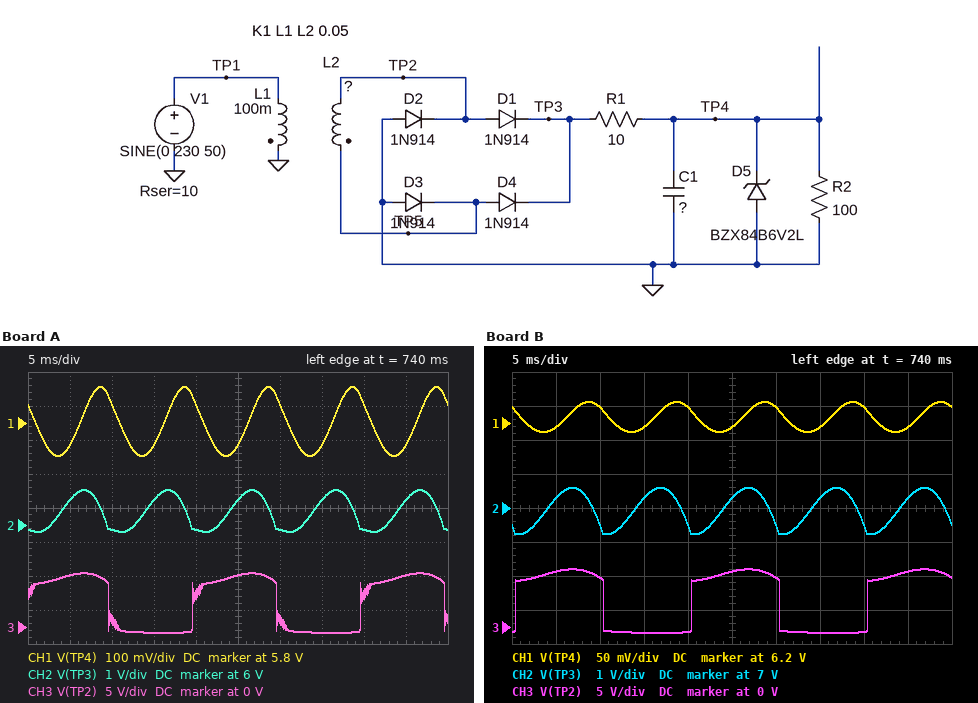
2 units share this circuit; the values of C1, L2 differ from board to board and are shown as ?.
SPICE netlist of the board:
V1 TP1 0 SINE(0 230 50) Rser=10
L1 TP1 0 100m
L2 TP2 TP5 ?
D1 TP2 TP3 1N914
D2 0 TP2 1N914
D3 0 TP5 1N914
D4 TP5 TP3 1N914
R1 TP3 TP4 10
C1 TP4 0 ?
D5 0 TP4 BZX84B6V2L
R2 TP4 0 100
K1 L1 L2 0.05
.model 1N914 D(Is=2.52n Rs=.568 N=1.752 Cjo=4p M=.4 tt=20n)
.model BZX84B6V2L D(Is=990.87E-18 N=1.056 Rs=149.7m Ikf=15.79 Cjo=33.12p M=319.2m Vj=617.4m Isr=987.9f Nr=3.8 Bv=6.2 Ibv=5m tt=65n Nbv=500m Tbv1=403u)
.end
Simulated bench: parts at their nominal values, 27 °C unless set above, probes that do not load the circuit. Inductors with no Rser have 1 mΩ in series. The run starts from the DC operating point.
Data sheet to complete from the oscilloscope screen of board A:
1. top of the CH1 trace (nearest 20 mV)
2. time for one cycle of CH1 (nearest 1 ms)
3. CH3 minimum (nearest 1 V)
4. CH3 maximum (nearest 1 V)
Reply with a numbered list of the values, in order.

1. 5.90 V
2. 10 ms
3. -1 V
4. 8 V
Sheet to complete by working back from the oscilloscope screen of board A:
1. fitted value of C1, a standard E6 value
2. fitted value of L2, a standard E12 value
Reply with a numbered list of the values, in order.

1. 1 mF
2. 120 mH
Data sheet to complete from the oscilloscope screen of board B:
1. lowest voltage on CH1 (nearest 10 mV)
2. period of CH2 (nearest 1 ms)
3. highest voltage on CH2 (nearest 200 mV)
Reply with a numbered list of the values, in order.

1. 6.19 V
2. 10 ms
3. 7.6 V
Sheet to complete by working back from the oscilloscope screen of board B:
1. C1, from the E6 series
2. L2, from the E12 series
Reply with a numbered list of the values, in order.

1. 4.7 mF
2. 180 mH
